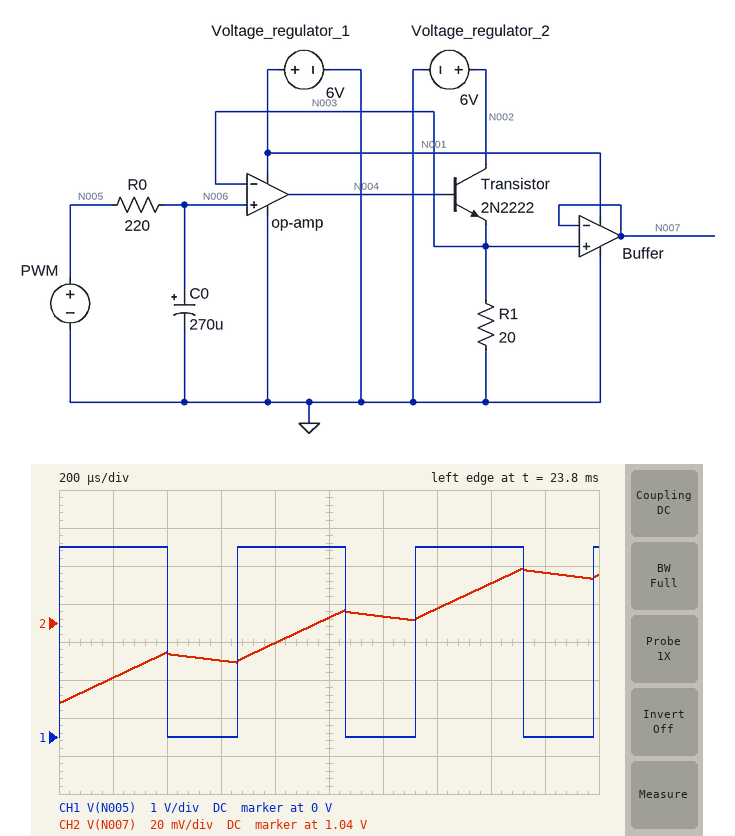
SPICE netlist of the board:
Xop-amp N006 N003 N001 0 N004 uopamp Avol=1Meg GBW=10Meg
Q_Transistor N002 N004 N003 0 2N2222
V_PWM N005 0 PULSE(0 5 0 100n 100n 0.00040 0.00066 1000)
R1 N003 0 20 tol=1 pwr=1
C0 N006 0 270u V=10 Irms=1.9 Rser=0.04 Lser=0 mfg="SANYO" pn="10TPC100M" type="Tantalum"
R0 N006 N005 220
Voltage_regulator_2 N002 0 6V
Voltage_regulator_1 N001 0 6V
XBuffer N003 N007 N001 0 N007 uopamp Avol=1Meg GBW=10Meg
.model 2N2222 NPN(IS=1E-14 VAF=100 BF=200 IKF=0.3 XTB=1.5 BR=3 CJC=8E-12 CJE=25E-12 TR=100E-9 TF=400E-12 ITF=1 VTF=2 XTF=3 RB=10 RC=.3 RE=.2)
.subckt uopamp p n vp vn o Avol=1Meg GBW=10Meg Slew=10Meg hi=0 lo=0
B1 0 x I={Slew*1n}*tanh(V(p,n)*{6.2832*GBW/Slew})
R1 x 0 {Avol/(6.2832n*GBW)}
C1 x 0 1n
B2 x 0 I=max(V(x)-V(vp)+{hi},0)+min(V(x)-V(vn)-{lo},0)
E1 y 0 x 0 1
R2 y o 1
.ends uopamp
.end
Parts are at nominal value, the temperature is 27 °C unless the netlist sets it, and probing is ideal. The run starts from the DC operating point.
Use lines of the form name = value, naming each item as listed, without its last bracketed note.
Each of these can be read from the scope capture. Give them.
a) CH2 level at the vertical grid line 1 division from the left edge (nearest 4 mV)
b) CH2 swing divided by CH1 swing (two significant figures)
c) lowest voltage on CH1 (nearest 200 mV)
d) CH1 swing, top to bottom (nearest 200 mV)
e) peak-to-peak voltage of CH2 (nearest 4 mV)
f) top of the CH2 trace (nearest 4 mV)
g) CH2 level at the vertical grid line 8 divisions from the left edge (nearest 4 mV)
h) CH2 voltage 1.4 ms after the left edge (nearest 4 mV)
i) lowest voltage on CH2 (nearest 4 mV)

CH2 level at the vertical grid line 1 division from the left edge = 1.012 V
CH2 swing divided by CH1 swing = 0.014
lowest voltage on CH1 = 0 V
CH1 swing, top to bottom = 5.0 V
peak-to-peak voltage of CH2 = 72 mV
top of the CH2 trace = 1.068 V
CH2 level at the vertical grid line 8 divisions from the left edge = 1.060 V
CH2 voltage 1.4 ms after the left edge = 1.048 V
lowest voltage on CH2 = 996 mV
